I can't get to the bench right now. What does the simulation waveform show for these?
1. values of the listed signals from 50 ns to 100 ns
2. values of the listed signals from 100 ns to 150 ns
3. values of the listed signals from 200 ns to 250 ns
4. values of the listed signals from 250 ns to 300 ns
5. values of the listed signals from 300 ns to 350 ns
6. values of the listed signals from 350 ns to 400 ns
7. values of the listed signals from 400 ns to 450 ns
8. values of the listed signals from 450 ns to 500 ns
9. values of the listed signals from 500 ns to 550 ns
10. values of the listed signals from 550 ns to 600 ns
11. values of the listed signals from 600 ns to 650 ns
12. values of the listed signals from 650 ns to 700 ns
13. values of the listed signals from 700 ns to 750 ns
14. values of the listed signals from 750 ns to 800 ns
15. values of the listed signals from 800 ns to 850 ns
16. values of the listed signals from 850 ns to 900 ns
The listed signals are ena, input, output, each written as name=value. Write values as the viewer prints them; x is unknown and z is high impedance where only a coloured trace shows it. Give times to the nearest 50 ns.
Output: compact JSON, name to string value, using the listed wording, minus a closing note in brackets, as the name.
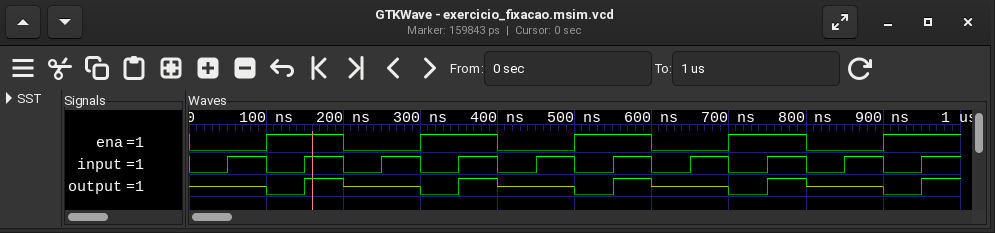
{"values of the listed signals from 50 ns to 100 ns": "ena=0, input=1, output=z", "values of the listed signals from 100 ns to 150 ns": "ena=1, input=0, output=0", "values of the listed signals from 200 ns to 250 ns": "ena=0, input=0, output=z", "values of the listed signals from 250 ns to 300 ns": "ena=0, input=1, output=z", "values of the listed signals from 300 ns to 350 ns": "ena=1, input=0, output=0", "values of the listed signals from 350 ns to 400 ns": "ena=1, input=1, output=1", "values of the listed signals from 400 ns to 450 ns": "ena=0, input=0, output=z", "values of the listed signals from 450 ns to 500 ns": "ena=0, input=1, output=z", "values of the listed signals from 500 ns to 550 ns": "ena=1, input=0, output=0", "values of the listed signals from 550 ns to 600 ns": "ena=1, input=1, output=1", "values of the listed signals from 600 ns to 650 ns": "ena=0, input=0, output=z", "values of the listed signals from 650 ns to 700 ns": "ena=0, input=1, output=z", "values of the listed signals from 700 ns to 750 ns": "ena=1, input=0, output=0", "values of the listed signals from 750 ns to 800 ns": "ena=1, input=1, output=1", "values of the listed signals from 800 ns to 850 ns": "ena=0, input=0, output=z", "values of the listed signals from 850 ns to 900 ns": "ena=0, input=1, output=z"}
